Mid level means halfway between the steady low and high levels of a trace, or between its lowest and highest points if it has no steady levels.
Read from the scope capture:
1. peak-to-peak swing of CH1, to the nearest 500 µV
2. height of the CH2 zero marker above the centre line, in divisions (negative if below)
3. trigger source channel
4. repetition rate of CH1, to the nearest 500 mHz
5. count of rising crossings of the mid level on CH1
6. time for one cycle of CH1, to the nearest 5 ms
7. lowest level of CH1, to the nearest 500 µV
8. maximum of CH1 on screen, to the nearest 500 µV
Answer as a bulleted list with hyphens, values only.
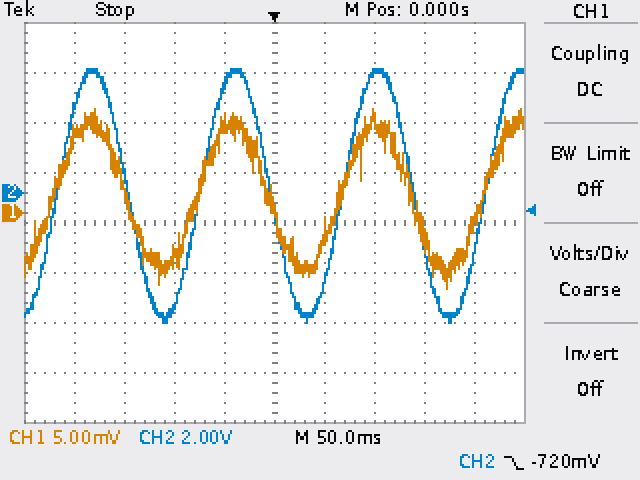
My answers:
- 18.0 mV
- +0.6 div
- CH2
- 7.0 Hz
- 4
- 145 ms
- -7.5 mV
- 10.5 mV
